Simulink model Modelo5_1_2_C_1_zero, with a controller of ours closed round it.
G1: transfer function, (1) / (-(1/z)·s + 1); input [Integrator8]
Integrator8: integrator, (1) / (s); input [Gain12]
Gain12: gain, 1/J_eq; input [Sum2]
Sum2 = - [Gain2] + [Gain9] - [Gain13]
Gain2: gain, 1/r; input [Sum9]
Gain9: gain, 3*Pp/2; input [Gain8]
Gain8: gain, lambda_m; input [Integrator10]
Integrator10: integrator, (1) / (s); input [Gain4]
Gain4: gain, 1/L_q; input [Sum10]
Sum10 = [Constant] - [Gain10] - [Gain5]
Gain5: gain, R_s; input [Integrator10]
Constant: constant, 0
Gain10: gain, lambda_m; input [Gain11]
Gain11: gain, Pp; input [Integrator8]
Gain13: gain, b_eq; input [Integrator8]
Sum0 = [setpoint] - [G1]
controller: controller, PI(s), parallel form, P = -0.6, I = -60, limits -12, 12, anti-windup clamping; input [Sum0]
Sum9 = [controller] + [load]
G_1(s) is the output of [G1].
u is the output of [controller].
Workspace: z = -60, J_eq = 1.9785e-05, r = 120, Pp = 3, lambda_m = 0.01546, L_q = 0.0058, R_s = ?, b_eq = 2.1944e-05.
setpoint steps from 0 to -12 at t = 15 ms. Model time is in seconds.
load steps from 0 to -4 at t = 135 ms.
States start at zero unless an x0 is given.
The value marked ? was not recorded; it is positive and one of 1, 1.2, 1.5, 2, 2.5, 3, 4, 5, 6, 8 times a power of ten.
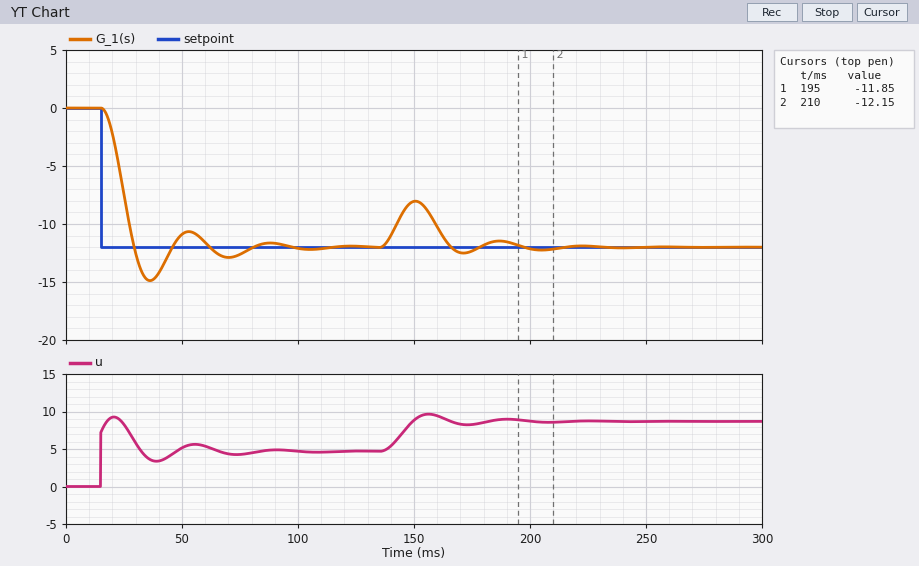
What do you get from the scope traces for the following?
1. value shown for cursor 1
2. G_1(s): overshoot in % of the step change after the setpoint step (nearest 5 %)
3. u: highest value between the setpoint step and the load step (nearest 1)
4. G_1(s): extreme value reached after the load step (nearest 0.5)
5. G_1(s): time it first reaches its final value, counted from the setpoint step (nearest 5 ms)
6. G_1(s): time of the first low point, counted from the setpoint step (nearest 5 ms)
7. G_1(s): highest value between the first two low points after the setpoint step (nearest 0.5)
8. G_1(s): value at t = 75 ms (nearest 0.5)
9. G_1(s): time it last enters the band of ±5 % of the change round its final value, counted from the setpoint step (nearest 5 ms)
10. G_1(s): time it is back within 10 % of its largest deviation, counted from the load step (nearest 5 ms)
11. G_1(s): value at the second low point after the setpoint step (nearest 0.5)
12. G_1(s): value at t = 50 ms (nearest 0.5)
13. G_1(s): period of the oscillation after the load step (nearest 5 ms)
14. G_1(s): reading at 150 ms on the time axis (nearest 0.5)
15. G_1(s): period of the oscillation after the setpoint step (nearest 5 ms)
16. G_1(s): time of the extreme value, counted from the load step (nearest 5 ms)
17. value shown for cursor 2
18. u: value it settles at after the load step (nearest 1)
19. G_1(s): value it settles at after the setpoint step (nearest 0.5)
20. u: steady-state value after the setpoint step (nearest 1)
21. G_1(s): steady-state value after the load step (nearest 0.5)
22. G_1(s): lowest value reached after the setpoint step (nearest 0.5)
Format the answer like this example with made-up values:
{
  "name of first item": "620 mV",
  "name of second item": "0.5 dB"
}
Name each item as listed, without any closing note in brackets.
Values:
{
  "value shown for cursor 1": "-11.85",
  "G_1(s): overshoot in % of the step change after the setpoint step": "25 %",
  "u: highest value between the setpoint step and the load step": "9",
  "G_1(s): extreme value reached after the load step": "-8.0",
  "G_1(s): time it first reaches its final value, counted from the setpoint step": "15 ms",
  "G_1(s): time of the first low point, counted from the setpoint step": "20 ms",
  "G_1(s): highest value between the first two low points after the setpoint step": "-10.5",
  "G_1(s): value at t = 75 ms": "-12.5",
  "G_1(s): time it last enters the band of ±5 % of the change round its final value, counted from the setpoint step": "60 ms",
  "G_1(s): time it is back within 10 % of its largest deviation, counted from the load step": "55 ms",
  "G_1(s): value at the second low point after the setpoint step": "-13.0",
  "G_1(s): value at t = 50 ms": "-11.0",
  "G_1(s): period of the oscillation after the load step": "35 ms",
  "G_1(s): reading at 150 ms on the time axis": "-8.0",
  "G_1(s): period of the oscillation after the setpoint step": "35 ms",
  "G_1(s): time of the extreme value, counted from the load step": "15 ms",
  "value shown for cursor 2": "-12.15",
  "u: value it settles at after the load step": "9",
  "G_1(s): value it settles at after the setpoint step": "-12.0",
  "u: steady-state value after the setpoint step": "5",
  "G_1(s): steady-state value after the load step": "-12.0",
  "G_1(s): lowest value reached after the setpoint step": "-15.0"
}
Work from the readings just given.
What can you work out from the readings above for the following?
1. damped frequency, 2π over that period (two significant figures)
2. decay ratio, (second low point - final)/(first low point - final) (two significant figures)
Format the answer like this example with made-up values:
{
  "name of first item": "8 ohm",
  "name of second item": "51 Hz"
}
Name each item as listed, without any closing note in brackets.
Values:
{
  "damped frequency, 2π over that period": "0.18 rad/ms",
  "decay ratio, (second low point - final)/(first low point - final)": "0.33"
}
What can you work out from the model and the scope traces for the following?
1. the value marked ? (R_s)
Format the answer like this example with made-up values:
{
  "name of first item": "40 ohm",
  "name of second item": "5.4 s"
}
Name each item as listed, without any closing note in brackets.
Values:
{
  "the value marked ?": "1"
}
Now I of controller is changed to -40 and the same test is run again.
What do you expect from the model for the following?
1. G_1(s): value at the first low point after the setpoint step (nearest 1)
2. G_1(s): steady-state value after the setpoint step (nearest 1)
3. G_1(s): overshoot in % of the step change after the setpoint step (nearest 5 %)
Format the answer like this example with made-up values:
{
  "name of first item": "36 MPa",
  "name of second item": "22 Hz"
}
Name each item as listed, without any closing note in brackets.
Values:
{
  "G_1(s): value at the first low point after the setpoint step": "-13",
  "G_1(s): steady-state value after the setpoint step": "-12",
  "G_1(s): overshoot in % of the step change after the setpoint step": "10 %"
}
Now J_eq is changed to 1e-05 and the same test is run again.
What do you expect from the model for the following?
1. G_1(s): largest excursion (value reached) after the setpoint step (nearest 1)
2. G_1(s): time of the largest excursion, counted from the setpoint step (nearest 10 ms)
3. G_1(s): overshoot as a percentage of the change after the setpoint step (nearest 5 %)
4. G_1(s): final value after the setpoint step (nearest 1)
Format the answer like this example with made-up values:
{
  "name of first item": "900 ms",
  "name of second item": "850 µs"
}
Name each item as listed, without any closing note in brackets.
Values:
{
  "G_1(s): largest excursion (value reached) after the setpoint step": "-13",
  "G_1(s): time of the largest excursion, counted from the setpoint step": "40 ms",
  "G_1(s): overshoot as a percentage of the change after the setpoint step": "10 %",
  "G_1(s): final value after the setpoint step": "-12"
}
